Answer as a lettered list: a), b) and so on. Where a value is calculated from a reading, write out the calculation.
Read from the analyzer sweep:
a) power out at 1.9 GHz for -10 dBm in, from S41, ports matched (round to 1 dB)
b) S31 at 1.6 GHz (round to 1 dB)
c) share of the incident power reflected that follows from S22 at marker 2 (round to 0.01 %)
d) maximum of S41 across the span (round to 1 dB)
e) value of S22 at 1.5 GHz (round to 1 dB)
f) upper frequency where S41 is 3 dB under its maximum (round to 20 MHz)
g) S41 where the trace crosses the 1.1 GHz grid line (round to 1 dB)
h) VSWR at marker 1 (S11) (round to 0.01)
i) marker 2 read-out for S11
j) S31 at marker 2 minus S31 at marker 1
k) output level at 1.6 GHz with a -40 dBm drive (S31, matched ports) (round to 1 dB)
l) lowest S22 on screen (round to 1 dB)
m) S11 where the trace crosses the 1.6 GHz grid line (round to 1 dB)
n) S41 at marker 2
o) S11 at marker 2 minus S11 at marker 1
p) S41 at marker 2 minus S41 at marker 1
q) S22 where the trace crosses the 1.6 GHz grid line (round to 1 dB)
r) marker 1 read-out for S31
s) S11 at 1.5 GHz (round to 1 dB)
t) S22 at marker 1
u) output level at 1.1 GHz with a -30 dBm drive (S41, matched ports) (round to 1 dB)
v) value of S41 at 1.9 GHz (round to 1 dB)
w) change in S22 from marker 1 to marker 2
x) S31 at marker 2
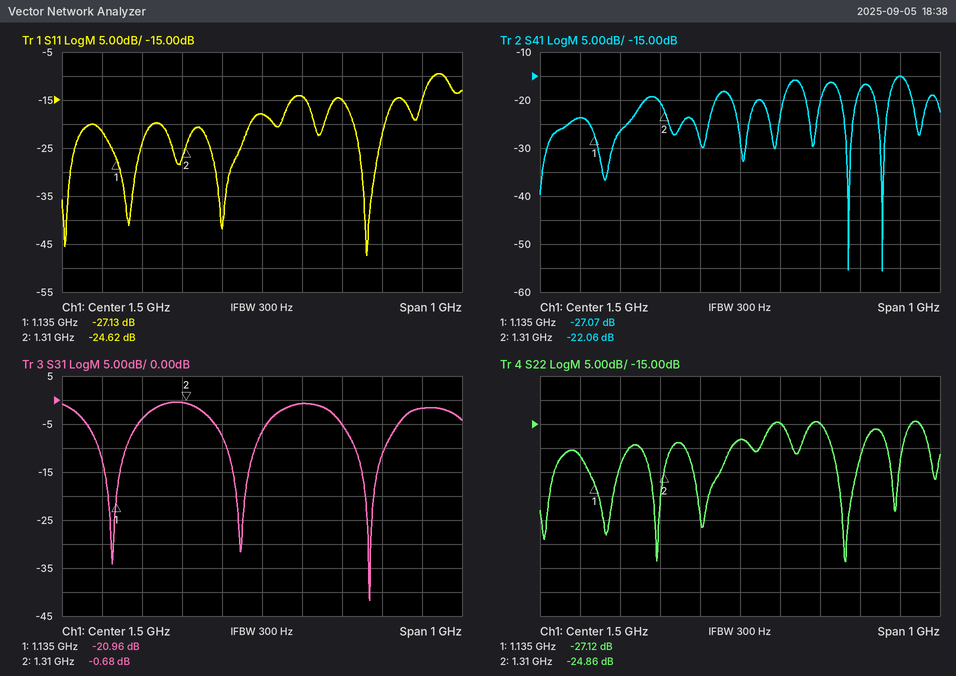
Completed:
a) -10 dBm + (-15 dB) = -25 dBm
b) -1 dB
c) 10^(-24.86/10) ≈ 0.33 %
d) -15 dB
e) -18 dB
f) 1.92 GHz
g) -24 dB
h) (1 + 0.0440)/(1 − 0.0440) ≈ 1.09
i) -24.62 dB
j) -0.68 − (-20.96) = 20.28 dB
k) -40 dBm + (-1 dB) = -41 dBm
l) -44 dB
m) -14 dB
n) -22.06 dB
o) -24.62 − (-27.13) = 2.51 dB
p) -22.06 − (-27.07) = 5.01 dB
q) -15 dB
r) -20.96 dB
s) -18 dB
t) -27.12 dB
u) -30 dBm + (-24 dB) = -54 dBm
v) -15 dB
w) -24.86 − (-27.12) = 2.26 dB
x) -0.68 dB
